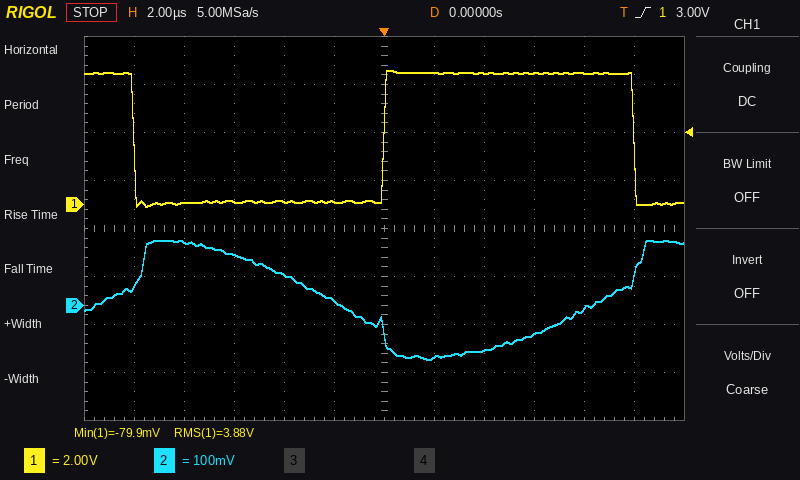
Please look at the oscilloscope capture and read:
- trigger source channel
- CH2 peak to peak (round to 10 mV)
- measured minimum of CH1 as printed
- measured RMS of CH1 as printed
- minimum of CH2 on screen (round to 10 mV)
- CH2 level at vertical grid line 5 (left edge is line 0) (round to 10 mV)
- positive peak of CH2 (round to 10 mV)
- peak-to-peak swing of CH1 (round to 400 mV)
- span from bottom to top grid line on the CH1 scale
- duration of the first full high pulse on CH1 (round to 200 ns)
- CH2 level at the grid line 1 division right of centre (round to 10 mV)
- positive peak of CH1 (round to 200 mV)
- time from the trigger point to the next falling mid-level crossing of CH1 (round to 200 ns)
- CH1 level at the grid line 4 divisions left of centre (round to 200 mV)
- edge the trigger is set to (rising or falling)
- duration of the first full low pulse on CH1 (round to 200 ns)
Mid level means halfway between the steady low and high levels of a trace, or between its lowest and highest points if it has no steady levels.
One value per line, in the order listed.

CH1
250 mV
-79.9 mV
3.88 V
-110 mV
10 mV
140 mV
5.6 V
16 V
10.0 µs
-110 mV
5.6 V
10.0 µs
0.0 V
rising
10.0 µs
